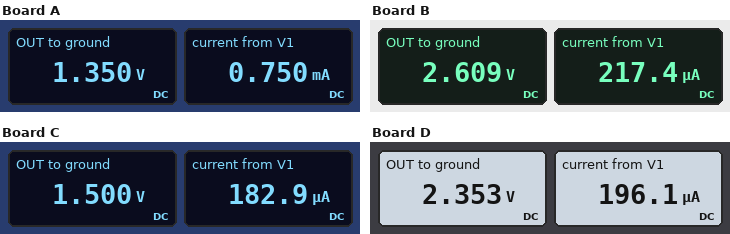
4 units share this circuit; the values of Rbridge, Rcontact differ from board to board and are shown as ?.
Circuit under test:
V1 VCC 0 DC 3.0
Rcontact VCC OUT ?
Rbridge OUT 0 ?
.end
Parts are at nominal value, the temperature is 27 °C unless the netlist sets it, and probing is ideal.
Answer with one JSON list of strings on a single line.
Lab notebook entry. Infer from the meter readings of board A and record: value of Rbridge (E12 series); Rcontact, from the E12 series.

["1.8 kΩ", "2.2 kΩ"]
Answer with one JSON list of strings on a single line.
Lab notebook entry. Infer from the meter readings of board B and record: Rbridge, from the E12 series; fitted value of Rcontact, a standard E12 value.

["12 kΩ", "1.8 kΩ"]
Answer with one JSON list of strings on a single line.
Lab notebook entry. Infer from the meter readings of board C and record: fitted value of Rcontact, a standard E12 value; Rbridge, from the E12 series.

["8.2 kΩ", "8.2 kΩ"]
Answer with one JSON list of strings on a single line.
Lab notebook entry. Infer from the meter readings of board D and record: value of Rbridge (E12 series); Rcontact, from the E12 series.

["12 kΩ", "3.3 kΩ"]
